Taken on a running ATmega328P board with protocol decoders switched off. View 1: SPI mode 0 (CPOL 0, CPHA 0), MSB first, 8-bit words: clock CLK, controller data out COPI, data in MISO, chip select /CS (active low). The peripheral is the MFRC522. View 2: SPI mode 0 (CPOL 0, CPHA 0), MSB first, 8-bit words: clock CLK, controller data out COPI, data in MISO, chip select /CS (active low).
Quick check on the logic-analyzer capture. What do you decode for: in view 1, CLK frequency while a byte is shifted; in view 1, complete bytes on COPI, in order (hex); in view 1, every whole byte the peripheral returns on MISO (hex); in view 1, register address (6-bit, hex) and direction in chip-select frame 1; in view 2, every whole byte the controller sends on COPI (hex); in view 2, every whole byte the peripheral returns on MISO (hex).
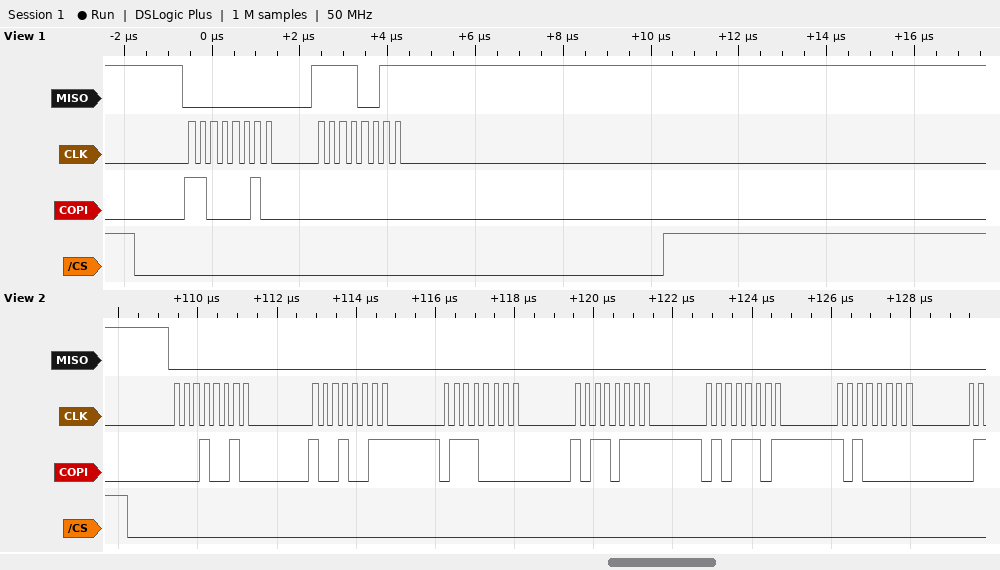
4 MHz
C2 00
00 F3
0x21 read
12 93 70 B7 5D A0
00 00 00 00 00 00
